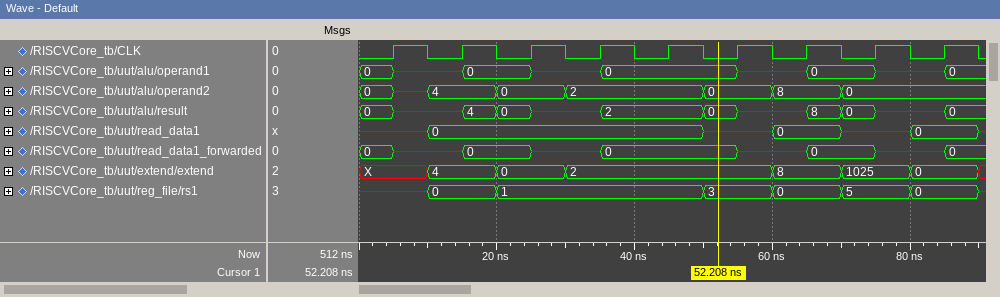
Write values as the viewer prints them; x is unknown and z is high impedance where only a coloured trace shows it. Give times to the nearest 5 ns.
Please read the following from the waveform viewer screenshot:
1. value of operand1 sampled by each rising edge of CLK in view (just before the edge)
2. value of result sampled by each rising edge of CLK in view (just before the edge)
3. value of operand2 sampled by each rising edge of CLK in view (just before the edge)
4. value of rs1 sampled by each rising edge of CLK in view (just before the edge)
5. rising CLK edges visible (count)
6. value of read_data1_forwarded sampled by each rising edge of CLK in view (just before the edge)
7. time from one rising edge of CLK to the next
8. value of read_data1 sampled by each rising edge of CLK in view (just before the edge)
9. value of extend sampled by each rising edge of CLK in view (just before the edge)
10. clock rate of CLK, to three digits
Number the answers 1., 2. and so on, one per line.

1. 0, x, 0, x, 0, 0, x, 0, x
2. 0, x, 0, x, 2, 0, x, 0, x
3. 0, 4, 0, 2, 2, 0, 8, 0, 0
4. x, 0, 1, 1, 1, 3, 0, 5, 0
5. 9
6. 0, x, 0, x, 0, 0, x, 0, x
7. 10 ns
8. x, 0, 0, 0, 0, x, 0, x, 0
9. X, 4, 0, 2, 2, 2, 8, 1025, 0
10. 100 MHz
